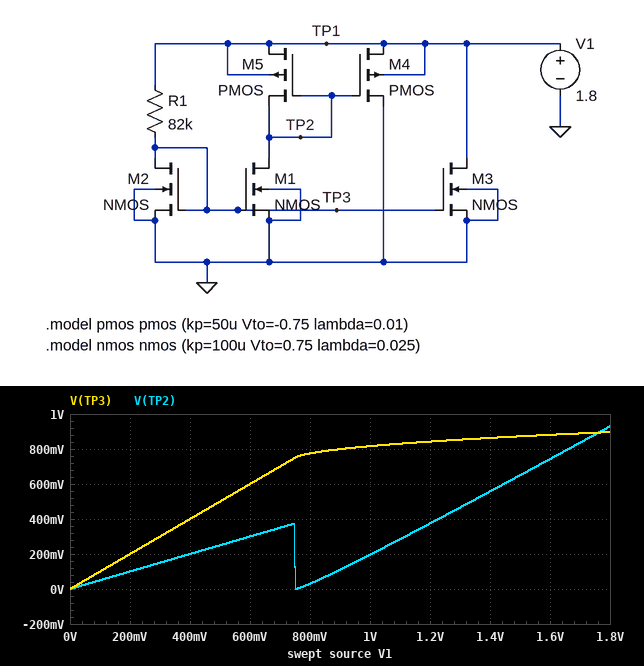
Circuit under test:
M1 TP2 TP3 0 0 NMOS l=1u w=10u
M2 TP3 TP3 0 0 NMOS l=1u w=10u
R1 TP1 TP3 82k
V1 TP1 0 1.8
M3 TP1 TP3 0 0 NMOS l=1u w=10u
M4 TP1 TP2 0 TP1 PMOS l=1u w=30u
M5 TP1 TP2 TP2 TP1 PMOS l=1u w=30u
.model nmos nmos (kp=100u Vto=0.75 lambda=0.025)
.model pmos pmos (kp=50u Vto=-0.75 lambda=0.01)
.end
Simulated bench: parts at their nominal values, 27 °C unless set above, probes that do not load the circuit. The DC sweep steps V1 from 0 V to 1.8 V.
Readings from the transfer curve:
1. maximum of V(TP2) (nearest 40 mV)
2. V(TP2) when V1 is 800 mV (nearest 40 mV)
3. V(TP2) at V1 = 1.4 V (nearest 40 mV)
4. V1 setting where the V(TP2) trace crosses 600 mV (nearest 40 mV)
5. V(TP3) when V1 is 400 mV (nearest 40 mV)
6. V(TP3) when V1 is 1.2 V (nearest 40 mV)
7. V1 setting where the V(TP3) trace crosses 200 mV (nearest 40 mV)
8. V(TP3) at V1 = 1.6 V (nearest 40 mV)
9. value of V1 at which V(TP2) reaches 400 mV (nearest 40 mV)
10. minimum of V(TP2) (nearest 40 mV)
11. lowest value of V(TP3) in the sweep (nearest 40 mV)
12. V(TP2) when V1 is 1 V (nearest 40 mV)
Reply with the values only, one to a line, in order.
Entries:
920 mV
40 mV
560 mV
1.44 V
400 mV
840 mV
200 mV
880 mV
1.24 V
0 V
0 V
200 mV
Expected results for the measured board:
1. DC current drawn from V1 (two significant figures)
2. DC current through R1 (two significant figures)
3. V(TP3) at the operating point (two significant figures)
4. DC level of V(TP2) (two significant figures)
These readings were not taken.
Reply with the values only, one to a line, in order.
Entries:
44 µA
11 µA
900 mV
930 mV
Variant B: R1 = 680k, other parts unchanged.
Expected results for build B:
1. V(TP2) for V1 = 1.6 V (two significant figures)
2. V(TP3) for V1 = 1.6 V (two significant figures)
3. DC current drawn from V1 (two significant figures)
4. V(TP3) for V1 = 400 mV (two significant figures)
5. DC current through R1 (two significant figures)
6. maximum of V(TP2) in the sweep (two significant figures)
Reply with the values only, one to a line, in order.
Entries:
810 mV
800 mV
5.9 µA
400 mV
1.5 µA
1.0 V
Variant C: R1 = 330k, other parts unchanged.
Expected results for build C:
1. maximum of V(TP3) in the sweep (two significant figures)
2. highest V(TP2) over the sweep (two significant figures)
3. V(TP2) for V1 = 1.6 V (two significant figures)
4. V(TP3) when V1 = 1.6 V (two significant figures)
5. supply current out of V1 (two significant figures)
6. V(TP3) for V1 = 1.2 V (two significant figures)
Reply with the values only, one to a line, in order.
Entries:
830 mV
990 mV
790 mV
820 mV
12 µA
800 mV
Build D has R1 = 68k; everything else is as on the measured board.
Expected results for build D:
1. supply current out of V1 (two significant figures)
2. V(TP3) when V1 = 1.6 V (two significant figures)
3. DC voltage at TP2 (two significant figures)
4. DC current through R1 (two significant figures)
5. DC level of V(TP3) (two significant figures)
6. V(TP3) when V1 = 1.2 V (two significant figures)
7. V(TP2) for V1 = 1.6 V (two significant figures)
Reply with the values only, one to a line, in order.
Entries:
53 µA
890 mV
920 mV
13 µA
910 mV
850 mV
730 mV
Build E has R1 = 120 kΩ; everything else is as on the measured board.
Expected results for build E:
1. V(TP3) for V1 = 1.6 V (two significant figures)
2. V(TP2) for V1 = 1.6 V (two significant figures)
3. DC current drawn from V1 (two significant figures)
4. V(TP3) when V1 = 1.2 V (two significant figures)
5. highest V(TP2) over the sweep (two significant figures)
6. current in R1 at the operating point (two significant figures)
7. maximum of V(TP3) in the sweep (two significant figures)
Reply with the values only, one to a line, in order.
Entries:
860 mV
760 mV
31 µA
830 mV
950 mV
7.7 µA
870 mV
